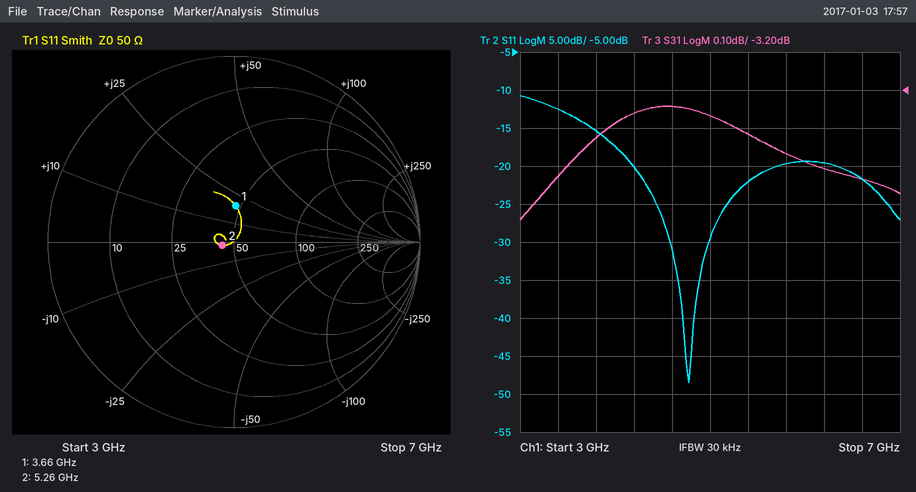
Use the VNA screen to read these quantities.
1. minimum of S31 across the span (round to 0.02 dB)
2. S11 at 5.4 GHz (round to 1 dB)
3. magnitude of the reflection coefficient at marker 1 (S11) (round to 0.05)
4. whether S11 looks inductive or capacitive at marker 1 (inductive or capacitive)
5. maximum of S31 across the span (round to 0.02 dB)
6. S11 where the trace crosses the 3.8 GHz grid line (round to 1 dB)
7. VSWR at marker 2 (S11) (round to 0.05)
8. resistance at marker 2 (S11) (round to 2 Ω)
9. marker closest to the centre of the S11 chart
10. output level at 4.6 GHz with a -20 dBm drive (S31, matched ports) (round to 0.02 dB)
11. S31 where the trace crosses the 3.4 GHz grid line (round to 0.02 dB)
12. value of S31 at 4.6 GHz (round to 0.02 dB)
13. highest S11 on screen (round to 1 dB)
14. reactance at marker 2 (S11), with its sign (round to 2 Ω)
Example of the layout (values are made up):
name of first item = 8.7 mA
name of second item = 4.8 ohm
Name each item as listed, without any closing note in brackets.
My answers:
minimum of S31 across the span = -3.54 dB
S11 at 5.4 GHz = -22 dB
magnitude of the reflection coefficient at marker 1 (S11) = 0.20
whether S11 looks inductive or capacitive at marker 1 = inductive
maximum of S31 across the span = -3.24 dB
S11 where the trace crosses the 3.8 GHz grid line = -15 dB
VSWR at marker 2 (S11) = 1.15
resistance at marker 2 (S11) = 44 Ω
marker closest to the centre of the S11 chart = marker 2
output level at 4.6 GHz with a -20 dBm drive (S31, matched ports) = -23.24 dBm
S31 where the trace crosses the 3.4 GHz grid line = -3.42 dB
value of S31 at 4.6 GHz = -3.24 dB
highest S11 on screen = -11 dB
reactance at marker 2 (S11), with its sign = -2 Ω
